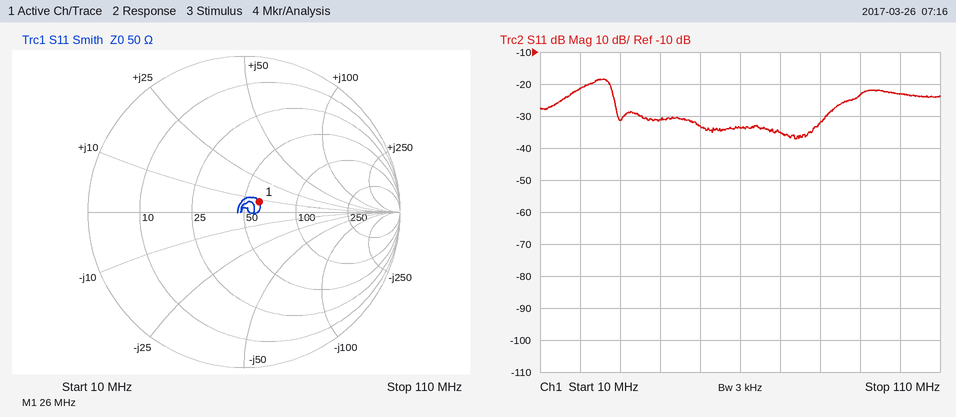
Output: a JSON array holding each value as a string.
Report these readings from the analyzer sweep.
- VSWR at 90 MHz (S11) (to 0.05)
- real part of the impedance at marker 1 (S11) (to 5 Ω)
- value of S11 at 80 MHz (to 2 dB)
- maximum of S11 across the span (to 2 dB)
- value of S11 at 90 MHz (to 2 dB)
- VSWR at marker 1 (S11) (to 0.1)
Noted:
["1.15", "60 Ω", "-32 dB", "-18 dB", "-24 dB", "1.3"]
